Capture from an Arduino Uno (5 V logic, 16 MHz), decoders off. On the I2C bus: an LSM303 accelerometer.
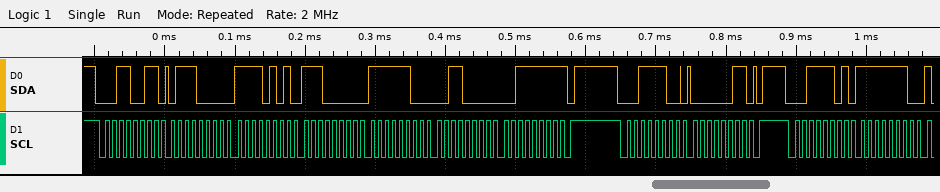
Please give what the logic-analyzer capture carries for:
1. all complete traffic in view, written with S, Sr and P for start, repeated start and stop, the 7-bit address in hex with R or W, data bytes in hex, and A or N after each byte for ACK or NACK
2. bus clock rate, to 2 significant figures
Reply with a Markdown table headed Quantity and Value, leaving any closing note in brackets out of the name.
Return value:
| Quantity | Value |
|---|---|
| all complete traffic in view, written with S, Sr and P for start, repeated start and stop, the 7-bit address in hex with R or W, data bytes in hex, and A or N after each byte for ACK or NACK | S 19R A 70 A F5 A E0 A FC A 30 A 3F N P S 1EW A 03 A P S 1ER A FE A |
| bus clock rate, to 2 significant figures | 100 kHz |
